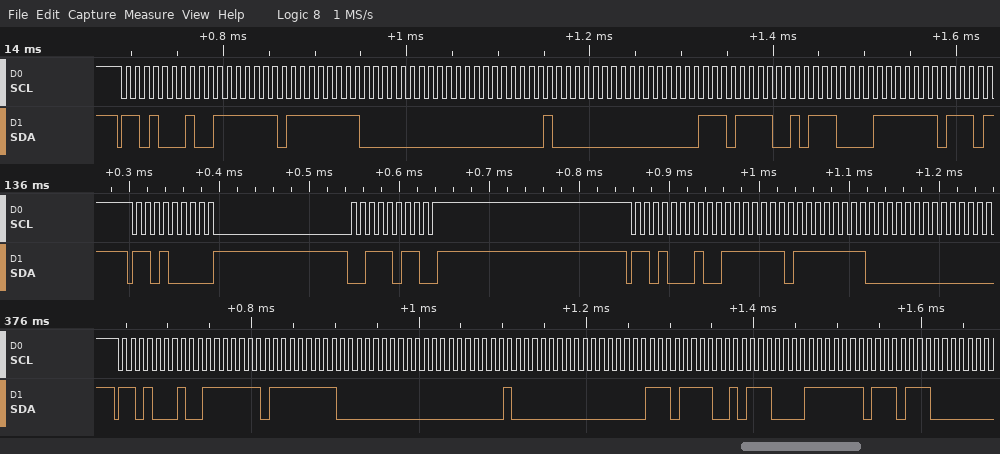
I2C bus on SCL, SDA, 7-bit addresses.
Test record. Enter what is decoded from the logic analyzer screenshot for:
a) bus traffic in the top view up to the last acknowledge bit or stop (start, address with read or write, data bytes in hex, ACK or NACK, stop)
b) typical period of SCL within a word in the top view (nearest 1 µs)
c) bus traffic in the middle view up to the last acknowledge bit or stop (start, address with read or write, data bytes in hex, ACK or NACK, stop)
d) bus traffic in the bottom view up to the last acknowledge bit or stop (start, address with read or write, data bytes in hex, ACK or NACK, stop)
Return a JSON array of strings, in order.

["start, address 68 read ACK, 7F ACK, FF ACK, 00 ACK, 00 ACK, 40 ACK, 00 ACK, EF ACK, 5C ACK, 7F ACK", "10 µs", "start, address 68 write ACK, 3B ACK, stop, start, address 68 read ACK, 7F ACK, FF ACK, 00 ACK", "start, address 68 read ACK, 7F ACK, FF ACK, 00 ACK, 00 ACK, 40 ACK, 00 ACK, EF ACK, 5C ACK, 7F ACK, EE ACK"]
